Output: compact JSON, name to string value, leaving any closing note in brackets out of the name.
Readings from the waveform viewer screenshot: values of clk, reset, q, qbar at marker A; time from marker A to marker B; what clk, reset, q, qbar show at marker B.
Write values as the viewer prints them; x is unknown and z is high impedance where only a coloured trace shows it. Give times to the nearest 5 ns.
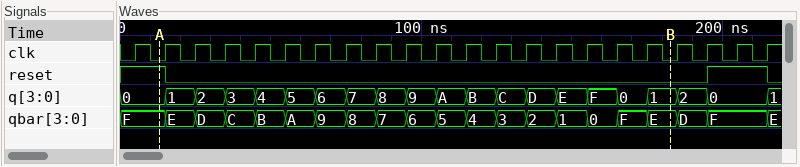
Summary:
{"values of clk, reset, q, qbar at marker A": "clk=0, reset=1, q=0, qbar=F", "time from marker A to marker B": "170 ns", "what clk, reset, q, qbar show at marker B": "clk=0, reset=0, q=1, qbar=E"}
